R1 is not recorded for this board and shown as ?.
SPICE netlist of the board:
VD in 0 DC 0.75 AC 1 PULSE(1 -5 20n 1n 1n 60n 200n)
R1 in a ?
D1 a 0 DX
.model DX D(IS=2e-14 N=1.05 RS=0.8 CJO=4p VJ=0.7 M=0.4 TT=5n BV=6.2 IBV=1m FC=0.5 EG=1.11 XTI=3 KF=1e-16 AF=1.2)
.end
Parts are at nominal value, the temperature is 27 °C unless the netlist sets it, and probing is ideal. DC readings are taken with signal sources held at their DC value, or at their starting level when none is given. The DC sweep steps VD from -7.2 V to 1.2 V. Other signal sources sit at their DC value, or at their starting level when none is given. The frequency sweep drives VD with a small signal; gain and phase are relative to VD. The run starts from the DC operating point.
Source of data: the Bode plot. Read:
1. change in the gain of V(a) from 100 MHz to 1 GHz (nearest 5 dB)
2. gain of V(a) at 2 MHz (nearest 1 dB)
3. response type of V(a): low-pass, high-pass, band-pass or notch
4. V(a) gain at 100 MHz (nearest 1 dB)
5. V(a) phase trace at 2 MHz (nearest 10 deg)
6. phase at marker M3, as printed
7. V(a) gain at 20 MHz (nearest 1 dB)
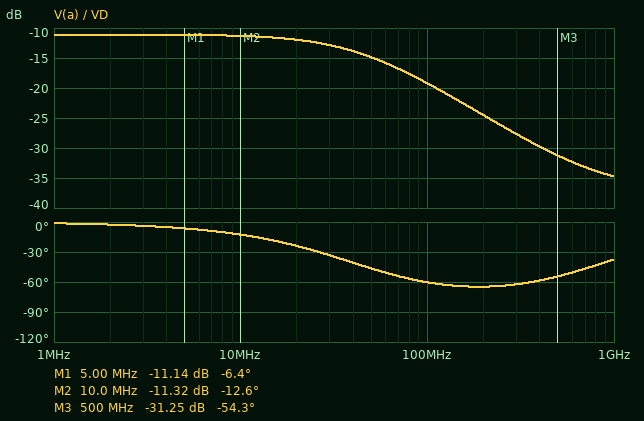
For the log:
-15 dB
-11 dB
low-pass
-19 dB
0 deg
-54.3 deg
-12 dB
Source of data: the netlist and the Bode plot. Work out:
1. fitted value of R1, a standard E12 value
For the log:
56 Ω
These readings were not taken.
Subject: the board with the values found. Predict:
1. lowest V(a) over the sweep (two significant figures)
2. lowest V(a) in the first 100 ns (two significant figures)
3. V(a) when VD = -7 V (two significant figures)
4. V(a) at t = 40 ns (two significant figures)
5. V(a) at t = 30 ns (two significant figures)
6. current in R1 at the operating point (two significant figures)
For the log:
-6.3 V
-5.0 V
-6.3 V
-5.0 V
-5.0 V
1.3 mA
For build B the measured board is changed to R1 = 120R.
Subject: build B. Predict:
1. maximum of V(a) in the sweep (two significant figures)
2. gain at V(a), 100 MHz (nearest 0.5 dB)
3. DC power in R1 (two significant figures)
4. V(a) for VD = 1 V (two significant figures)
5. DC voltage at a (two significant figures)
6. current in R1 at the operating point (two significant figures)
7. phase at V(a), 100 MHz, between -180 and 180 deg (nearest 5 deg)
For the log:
710 mV
-21.0 dB
65 µW
700 mV
660 mV
740 µA
-65 deg
